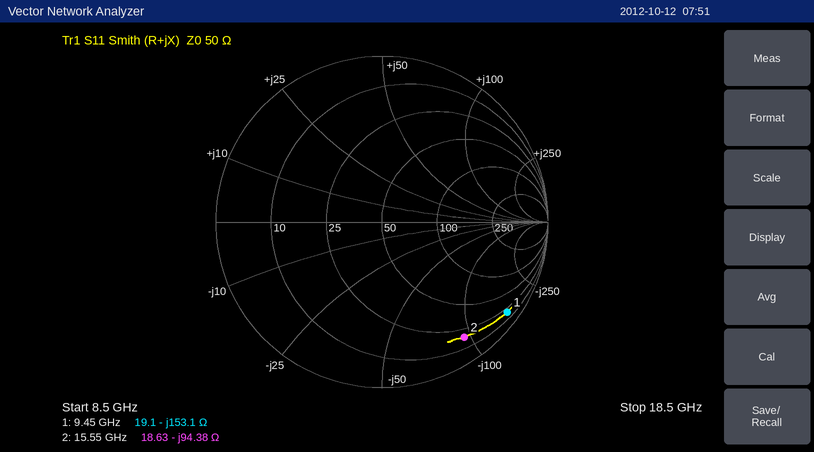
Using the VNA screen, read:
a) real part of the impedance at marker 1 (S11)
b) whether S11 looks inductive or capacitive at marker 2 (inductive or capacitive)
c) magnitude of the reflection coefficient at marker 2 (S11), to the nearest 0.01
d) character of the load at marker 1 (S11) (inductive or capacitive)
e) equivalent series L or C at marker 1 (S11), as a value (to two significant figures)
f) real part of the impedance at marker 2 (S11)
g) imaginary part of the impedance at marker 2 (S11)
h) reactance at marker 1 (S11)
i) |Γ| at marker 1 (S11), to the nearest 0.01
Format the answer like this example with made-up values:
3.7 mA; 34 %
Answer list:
19.1 Ω; capacitive; 0.85; capacitive; 110 fF; 18.63 Ω; -94.38 Ω; -153.1 Ω; 0.93
